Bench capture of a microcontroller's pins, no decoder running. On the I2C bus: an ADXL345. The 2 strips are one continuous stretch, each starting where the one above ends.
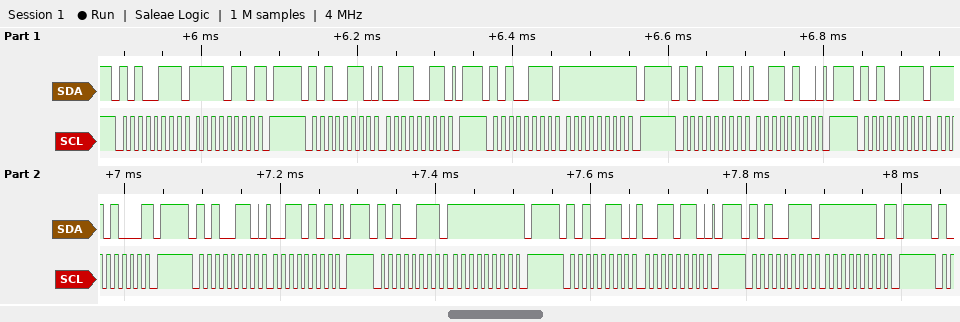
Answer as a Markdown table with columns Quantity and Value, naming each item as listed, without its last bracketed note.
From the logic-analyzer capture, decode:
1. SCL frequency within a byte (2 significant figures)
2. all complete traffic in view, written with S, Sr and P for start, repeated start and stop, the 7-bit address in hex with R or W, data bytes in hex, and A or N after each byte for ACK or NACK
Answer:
| Quantity | Value |
|---|---|
| SCL frequency within a byte | 100 kHz |
| all complete traffic in view, written with S, Sr and P for start, repeated start and stop, the 7-bit address in hex with R or W, data bytes in hex, and A or N after each byte for ACK or NACK | S 53R A F6 N P S 53W A 33 A P S 53R A FF N P S 53W A 34 A P S 53R A E8 N P S 53W A 35 A P S 53R A FF N P S 53W A 36 A P S 53R A FE N P |
